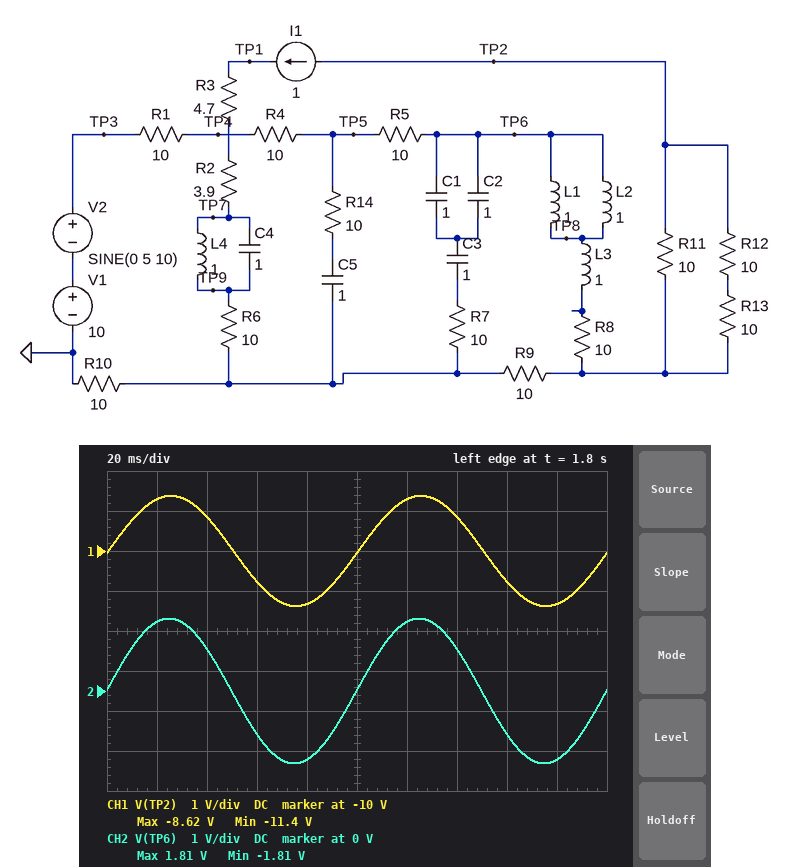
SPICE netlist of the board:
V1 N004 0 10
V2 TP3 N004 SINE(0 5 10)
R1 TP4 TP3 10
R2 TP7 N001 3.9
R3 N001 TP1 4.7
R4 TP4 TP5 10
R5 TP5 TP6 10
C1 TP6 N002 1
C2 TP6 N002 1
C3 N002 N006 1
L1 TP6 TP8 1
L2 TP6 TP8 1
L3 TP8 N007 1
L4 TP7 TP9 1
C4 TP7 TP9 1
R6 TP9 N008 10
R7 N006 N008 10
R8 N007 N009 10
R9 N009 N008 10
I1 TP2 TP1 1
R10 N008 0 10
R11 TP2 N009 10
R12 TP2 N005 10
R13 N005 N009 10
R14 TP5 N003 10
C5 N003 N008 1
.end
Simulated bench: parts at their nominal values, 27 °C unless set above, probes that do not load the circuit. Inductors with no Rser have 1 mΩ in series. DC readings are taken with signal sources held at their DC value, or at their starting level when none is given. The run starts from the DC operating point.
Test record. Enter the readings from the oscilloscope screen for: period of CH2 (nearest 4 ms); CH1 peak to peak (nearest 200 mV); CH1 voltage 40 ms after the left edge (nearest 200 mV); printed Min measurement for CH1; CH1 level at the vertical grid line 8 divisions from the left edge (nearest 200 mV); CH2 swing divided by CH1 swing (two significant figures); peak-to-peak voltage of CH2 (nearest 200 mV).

100 ms
2.8 V
-9.2 V
-11.4 V
-10.8 V
1.3
3.6 V
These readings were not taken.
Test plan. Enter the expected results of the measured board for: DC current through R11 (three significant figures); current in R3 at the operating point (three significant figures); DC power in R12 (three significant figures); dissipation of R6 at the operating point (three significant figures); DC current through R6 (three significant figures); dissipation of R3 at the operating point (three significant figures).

667 mA
1.00 A
1.11 W
10.0 W
1.00 A
4.70 W
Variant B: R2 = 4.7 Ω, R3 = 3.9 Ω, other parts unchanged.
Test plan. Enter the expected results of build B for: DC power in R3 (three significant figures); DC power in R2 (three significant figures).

3.90 W
4.70 W
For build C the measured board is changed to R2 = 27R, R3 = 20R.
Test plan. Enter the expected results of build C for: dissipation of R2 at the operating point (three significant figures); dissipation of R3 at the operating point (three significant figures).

27.0 W
20.0 W
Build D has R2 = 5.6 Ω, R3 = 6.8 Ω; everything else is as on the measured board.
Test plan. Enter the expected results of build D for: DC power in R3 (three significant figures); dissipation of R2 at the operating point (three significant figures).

6.80 W
5.60 W
